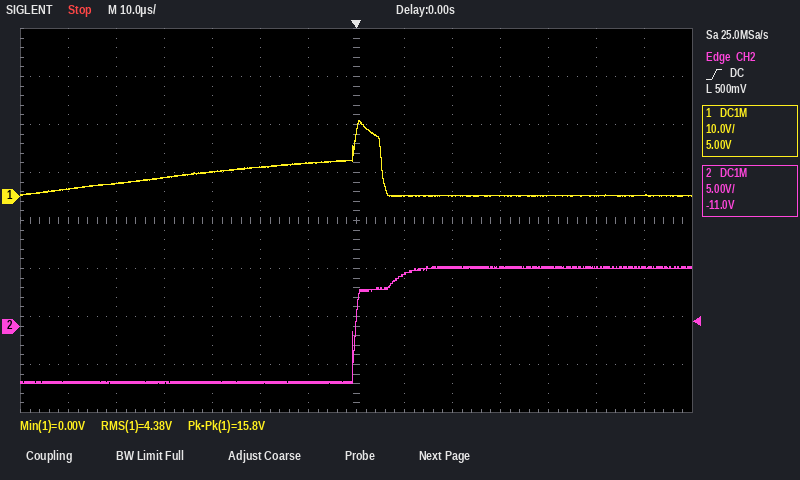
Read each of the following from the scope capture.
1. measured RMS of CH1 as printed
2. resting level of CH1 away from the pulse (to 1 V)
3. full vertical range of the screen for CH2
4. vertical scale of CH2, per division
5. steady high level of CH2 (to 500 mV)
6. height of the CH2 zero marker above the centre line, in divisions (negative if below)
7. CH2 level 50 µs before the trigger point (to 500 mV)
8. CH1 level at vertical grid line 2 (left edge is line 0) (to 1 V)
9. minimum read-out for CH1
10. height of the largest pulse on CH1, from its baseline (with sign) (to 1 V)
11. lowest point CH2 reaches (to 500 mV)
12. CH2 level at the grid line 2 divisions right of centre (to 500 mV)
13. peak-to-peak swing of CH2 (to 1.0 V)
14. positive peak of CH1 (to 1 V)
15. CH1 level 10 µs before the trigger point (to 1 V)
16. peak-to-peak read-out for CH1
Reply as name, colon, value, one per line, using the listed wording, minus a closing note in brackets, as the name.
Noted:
measured RMS of CH1 as printed: 4.38 V
resting level of CH1 away from the pulse: 0 V
full vertical range of the screen for CH2: 40 V
vertical scale of CH2, per division: 5 V
steady high level of CH2: 6.0 V
height of the CH2 zero marker above the centre line, in divisions: -2.2 div
CH2 level 50 µs before the trigger point: -6.0 V
CH1 level at vertical grid line 2 (left edge is line 0): 3 V
minimum read-out for CH1: 0.00 V
height of the largest pulse on CH1, from its baseline (with sign): +16 V
lowest point CH2 reaches: -6.0 V
CH2 level at the grid line 2 divisions right of centre: 6.0 V
peak-to-peak swing of CH2: 12.0 V
positive peak of CH1: 16 V
CH1 level 10 µs before the trigger point: 7 V
peak-to-peak read-out for CH1: 15.8 V
